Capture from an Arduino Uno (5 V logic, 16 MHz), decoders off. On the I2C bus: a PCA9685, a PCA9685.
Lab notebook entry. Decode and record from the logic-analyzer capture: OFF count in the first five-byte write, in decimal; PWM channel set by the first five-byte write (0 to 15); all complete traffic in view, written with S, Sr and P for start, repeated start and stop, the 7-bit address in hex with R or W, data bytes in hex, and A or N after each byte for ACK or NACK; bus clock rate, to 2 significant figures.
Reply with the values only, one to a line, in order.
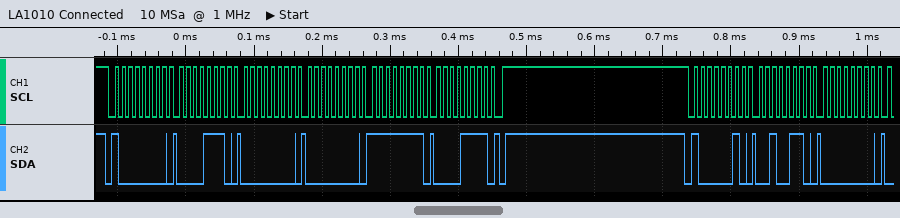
4095
2
S 40W A 0E A 00 A 00 A FF A 0F A P S 41W A 26 A 00 A
100 kHz
